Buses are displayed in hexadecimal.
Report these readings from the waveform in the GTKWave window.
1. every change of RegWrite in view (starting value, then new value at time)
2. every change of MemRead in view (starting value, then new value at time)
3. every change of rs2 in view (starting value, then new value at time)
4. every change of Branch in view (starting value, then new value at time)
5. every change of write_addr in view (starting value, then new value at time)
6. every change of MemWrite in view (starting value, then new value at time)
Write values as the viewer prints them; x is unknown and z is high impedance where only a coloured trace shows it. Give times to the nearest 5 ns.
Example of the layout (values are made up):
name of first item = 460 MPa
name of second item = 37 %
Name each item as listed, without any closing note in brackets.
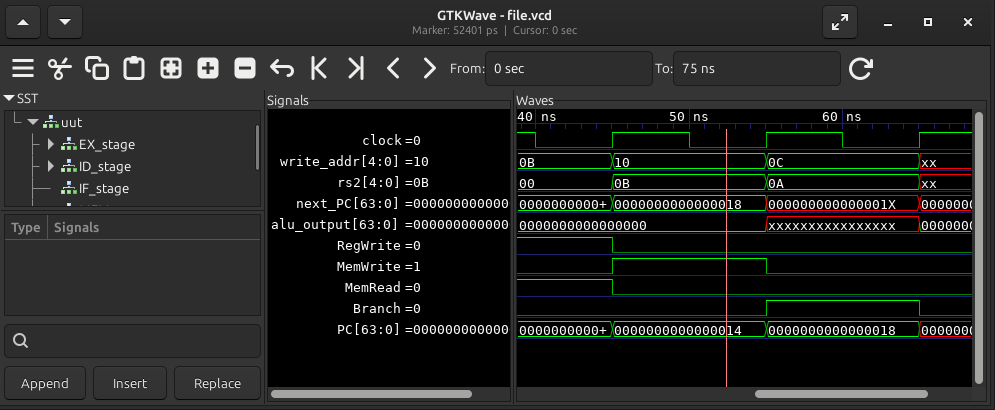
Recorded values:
every change of RegWrite in view = 1, 0 at 45 ns
every change of MemRead in view = 1, 0 at 45 ns
every change of rs2 in view = 00, 0B at 45 ns, 0A at 55 ns, xx at 65 ns
every change of Branch in view = 0, 1 at 55 ns, 0 at 65 ns
every change of write_addr in view = 0B, 10 at 45 ns, 0C at 55 ns, xx at 65 ns
every change of MemWrite in view = 0, 1 at 45 ns, 0 at 55 ns
